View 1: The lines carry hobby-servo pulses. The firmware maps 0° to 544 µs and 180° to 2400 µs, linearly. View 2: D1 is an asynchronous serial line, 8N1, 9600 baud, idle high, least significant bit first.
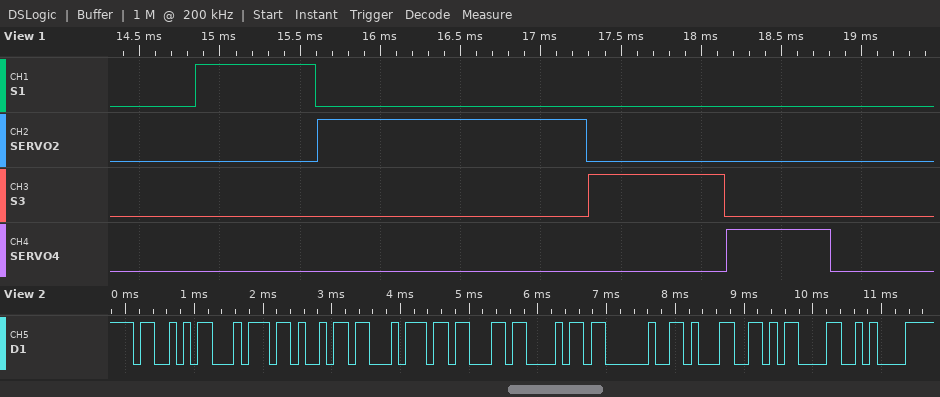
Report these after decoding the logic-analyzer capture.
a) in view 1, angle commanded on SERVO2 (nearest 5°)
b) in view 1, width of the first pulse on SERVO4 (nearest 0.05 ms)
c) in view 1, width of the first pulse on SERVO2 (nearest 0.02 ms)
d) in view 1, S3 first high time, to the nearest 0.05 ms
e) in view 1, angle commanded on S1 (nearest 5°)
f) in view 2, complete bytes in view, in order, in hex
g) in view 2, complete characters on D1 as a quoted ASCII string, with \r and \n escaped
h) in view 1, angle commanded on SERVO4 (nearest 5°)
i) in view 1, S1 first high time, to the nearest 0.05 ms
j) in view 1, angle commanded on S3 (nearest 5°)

110°
0.65 ms
1.68 ms
0.85 ms
20°
0x53 0x74 0x69 0x74 0x63 0x68 0x20 0x31 0x0D 0x0A
"Stitch 1\r\n"
10°
0.75 ms
30°
